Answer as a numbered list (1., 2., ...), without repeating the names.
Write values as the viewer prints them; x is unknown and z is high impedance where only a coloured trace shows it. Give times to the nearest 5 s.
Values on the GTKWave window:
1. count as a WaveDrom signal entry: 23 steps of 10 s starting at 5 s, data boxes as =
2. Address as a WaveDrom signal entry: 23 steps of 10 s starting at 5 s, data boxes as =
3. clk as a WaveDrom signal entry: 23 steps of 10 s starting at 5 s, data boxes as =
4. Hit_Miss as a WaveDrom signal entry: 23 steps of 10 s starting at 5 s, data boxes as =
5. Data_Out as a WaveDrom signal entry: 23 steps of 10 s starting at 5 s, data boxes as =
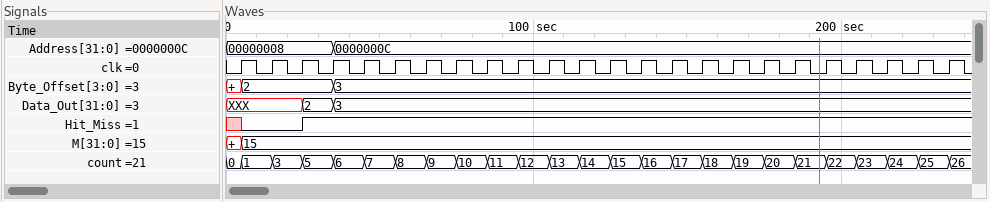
1. {name: 'count', wave: '=======================', data: '1 3 5 6 7 8 9 10 11 12 13 14 15 16 17 18 19 20 21 22 23 24 25'}
2. {name: 'Address', wave: '=..=...................', data: '00000008 0000000C'}
3. {name: 'clk', wave: 'p......................'}
4. {name: 'Hit_Miss', wave: '0.1....................'}
5. {name: 'Data_Out', wave: 'x.==...................', data: '2 3'}
